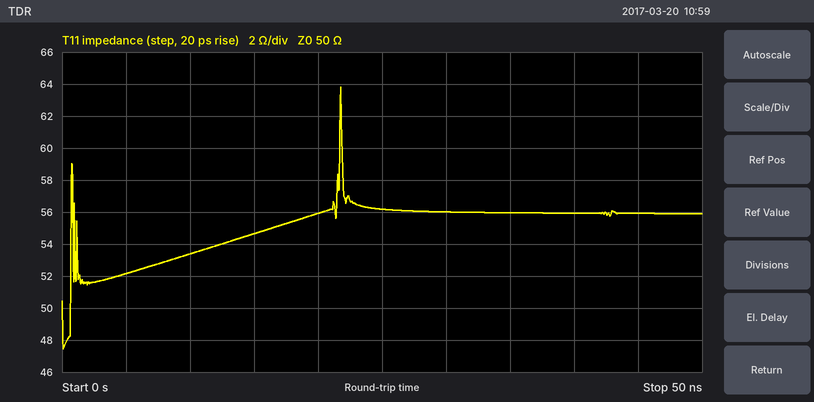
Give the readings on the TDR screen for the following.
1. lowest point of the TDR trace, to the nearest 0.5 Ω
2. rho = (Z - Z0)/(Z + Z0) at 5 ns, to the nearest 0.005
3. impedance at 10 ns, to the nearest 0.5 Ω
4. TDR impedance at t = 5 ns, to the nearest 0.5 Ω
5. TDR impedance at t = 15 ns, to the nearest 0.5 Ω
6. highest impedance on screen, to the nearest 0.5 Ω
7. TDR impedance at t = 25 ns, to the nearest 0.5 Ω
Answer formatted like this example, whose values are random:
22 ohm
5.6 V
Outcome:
47.5 Ω
+0.020
53.5 Ω
52.0 Ω
54.5 Ω
64.0 Ω
56.0 Ω
